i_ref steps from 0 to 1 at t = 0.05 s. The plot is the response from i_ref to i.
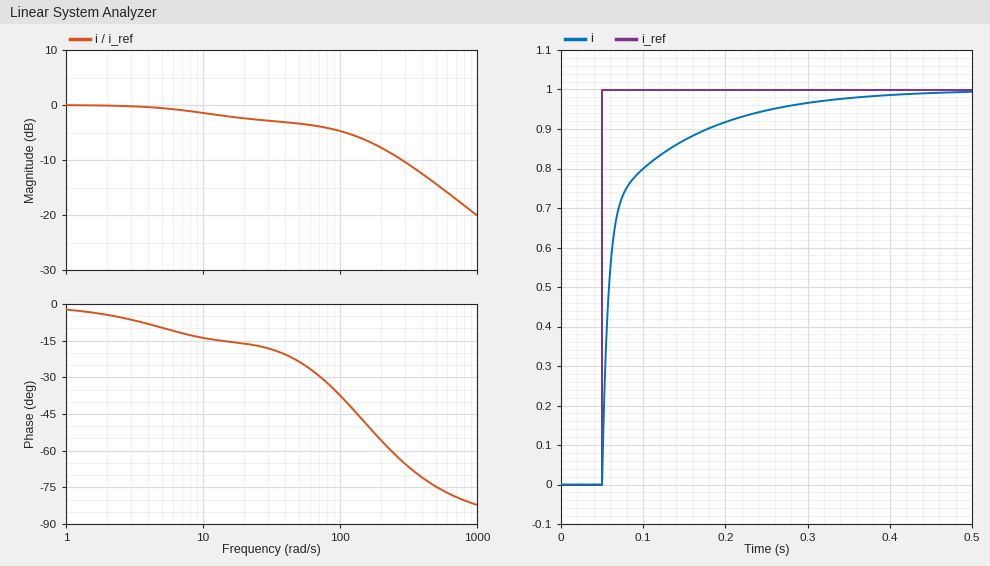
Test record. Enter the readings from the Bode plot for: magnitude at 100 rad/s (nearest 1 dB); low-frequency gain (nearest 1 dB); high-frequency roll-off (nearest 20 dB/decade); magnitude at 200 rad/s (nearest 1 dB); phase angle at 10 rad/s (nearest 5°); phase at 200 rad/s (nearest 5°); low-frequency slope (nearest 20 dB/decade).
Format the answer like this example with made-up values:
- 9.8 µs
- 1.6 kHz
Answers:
- -5 dB
- 0 dB
- -20 dB/decade
- -8 dB
- -15°
- -55°
- 0 dB/decade
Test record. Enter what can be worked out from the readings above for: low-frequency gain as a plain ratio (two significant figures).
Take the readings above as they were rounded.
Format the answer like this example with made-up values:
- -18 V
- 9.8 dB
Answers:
- 1.0
